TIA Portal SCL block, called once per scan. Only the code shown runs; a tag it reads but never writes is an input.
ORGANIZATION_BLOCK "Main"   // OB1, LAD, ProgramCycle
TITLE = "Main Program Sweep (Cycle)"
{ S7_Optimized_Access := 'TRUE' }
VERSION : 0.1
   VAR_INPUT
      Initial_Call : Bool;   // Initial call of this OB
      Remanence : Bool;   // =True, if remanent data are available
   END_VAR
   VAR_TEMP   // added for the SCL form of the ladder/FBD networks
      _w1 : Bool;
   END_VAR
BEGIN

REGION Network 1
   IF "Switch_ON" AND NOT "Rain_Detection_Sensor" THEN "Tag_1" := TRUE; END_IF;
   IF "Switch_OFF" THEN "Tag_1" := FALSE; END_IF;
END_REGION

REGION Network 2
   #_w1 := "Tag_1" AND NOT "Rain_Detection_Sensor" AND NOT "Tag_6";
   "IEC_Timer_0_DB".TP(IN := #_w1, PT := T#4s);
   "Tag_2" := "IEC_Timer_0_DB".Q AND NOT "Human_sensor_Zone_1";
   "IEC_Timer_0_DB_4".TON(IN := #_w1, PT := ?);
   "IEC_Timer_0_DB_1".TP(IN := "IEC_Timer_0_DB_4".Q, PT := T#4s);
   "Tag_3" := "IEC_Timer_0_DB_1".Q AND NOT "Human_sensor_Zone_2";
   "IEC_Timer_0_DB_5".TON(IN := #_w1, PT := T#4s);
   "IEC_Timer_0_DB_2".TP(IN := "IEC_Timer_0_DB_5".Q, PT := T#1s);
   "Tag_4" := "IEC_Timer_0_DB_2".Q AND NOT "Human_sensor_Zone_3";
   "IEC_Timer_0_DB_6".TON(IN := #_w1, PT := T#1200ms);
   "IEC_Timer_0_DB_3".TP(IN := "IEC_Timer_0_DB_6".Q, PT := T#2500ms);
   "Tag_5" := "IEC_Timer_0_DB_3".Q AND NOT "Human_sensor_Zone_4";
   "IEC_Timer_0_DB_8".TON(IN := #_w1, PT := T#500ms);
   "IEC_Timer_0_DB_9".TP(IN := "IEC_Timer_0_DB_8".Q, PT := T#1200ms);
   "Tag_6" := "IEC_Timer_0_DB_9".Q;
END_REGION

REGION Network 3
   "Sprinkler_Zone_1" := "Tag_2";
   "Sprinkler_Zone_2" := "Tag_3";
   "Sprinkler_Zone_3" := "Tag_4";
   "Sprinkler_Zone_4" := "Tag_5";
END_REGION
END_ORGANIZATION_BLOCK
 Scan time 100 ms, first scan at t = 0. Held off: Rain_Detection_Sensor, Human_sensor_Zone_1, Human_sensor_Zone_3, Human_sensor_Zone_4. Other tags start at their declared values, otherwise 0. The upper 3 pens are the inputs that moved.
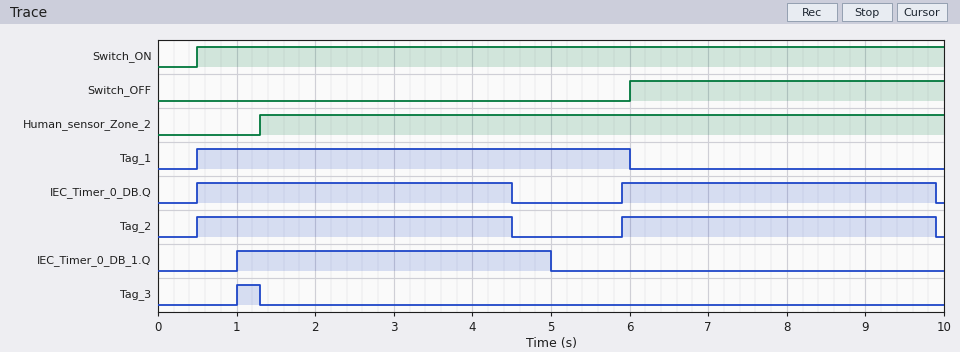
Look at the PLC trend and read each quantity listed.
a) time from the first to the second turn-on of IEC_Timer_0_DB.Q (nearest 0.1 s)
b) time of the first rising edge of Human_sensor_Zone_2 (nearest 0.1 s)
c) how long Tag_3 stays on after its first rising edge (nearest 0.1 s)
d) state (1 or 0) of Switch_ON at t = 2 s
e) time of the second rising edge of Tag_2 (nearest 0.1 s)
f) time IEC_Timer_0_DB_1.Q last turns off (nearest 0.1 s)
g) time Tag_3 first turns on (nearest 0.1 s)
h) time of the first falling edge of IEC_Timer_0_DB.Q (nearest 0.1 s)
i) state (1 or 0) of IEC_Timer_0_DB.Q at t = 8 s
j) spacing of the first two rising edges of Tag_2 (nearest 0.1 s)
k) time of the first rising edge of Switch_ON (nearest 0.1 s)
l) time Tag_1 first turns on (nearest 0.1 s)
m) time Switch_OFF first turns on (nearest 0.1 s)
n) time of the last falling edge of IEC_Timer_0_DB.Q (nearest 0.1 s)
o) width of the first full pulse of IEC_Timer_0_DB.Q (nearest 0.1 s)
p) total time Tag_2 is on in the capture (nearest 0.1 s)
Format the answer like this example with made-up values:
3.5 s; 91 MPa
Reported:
5.4 s; 1.3 s; 0.3 s; 1; 5.9 s; 5.0 s; 1.0 s; 4.5 s; 1; 5.4 s; 0.5 s; 0.5 s; 6.0 s; 9.9 s; 4.0 s; 8.0 s
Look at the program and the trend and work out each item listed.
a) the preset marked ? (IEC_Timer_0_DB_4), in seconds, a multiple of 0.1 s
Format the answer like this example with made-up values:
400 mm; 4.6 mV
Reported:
0.5 s
